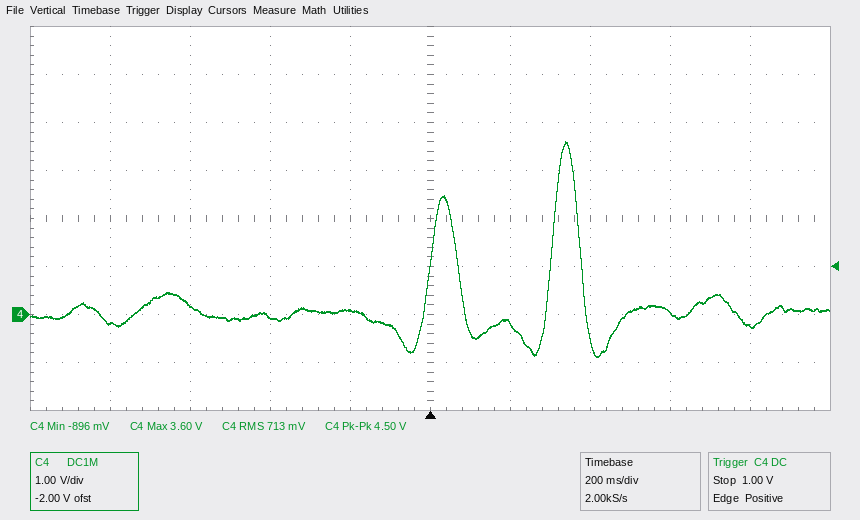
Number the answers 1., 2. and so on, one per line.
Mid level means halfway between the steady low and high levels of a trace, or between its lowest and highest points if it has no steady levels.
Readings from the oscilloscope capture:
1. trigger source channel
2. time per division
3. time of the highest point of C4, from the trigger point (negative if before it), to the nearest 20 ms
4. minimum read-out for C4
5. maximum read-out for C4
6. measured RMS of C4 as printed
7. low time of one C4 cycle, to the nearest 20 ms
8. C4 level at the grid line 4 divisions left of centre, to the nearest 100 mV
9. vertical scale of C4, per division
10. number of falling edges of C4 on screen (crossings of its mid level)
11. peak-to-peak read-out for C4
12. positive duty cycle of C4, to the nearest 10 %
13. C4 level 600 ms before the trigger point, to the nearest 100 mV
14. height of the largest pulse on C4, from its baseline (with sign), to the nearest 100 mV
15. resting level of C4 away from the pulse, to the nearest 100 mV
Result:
1. C4
2. 200 ms
3. +340 ms
4. -896 mV
5. 3.60 V
6. 713 mV
7. 240 ms
8. -200 mV
9. 1 V
10. 2
11. 4.50 V
12. 20 %
13. 200 mV
14. +3.6 V
15. 0.0 V
